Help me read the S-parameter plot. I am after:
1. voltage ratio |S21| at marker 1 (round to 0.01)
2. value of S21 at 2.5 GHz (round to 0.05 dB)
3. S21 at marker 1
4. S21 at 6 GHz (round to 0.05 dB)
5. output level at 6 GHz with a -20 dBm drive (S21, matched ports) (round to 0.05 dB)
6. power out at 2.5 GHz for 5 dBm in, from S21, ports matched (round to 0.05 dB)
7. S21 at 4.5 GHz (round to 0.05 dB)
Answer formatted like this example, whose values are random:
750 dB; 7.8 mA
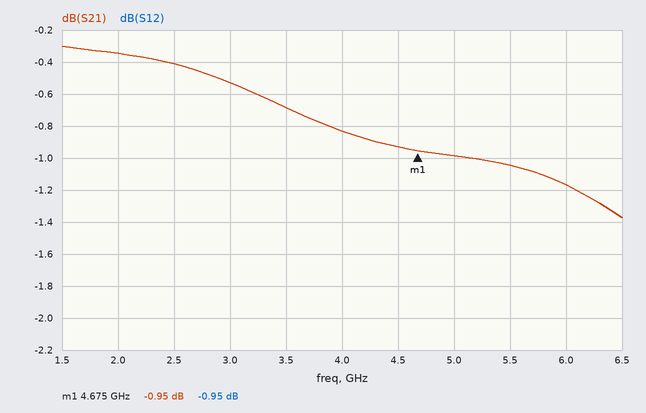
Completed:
0.90; -0.40 dB; -0.95 dB; -1.15 dB; -21.15 dBm; 4.60 dBm; -0.95 dB
